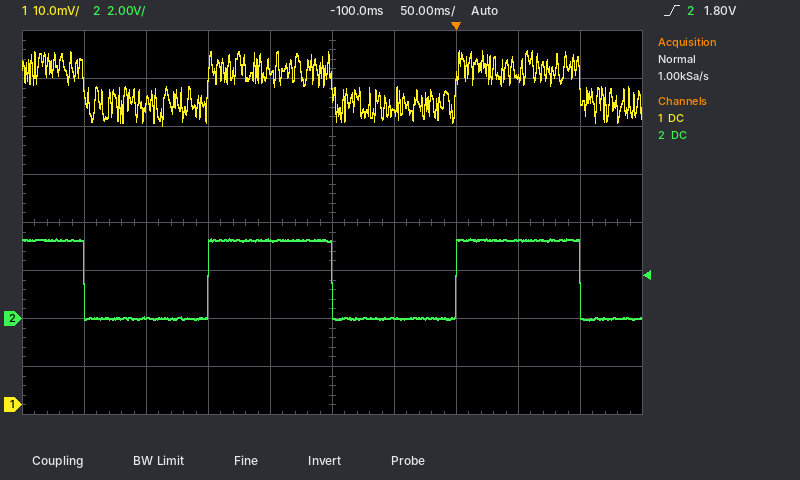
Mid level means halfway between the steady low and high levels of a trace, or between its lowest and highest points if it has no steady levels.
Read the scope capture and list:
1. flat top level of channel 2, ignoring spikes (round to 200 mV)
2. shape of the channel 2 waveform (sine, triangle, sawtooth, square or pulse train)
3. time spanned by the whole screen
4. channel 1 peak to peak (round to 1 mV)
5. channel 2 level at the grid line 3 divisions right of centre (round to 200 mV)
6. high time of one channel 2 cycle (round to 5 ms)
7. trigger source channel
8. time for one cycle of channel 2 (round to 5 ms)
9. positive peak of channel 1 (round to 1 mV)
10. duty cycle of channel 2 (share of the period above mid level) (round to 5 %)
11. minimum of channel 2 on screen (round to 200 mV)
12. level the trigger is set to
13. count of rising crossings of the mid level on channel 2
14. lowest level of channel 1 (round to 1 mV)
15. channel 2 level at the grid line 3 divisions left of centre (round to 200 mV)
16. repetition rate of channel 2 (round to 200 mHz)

3.2 V
square
500 ms
16 mV
3.2 V
100 ms
channel 2
200 ms
74 mV
50 %
0.0 V
1.80 V
2
58 mV
0.0 V
5.0 Hz
